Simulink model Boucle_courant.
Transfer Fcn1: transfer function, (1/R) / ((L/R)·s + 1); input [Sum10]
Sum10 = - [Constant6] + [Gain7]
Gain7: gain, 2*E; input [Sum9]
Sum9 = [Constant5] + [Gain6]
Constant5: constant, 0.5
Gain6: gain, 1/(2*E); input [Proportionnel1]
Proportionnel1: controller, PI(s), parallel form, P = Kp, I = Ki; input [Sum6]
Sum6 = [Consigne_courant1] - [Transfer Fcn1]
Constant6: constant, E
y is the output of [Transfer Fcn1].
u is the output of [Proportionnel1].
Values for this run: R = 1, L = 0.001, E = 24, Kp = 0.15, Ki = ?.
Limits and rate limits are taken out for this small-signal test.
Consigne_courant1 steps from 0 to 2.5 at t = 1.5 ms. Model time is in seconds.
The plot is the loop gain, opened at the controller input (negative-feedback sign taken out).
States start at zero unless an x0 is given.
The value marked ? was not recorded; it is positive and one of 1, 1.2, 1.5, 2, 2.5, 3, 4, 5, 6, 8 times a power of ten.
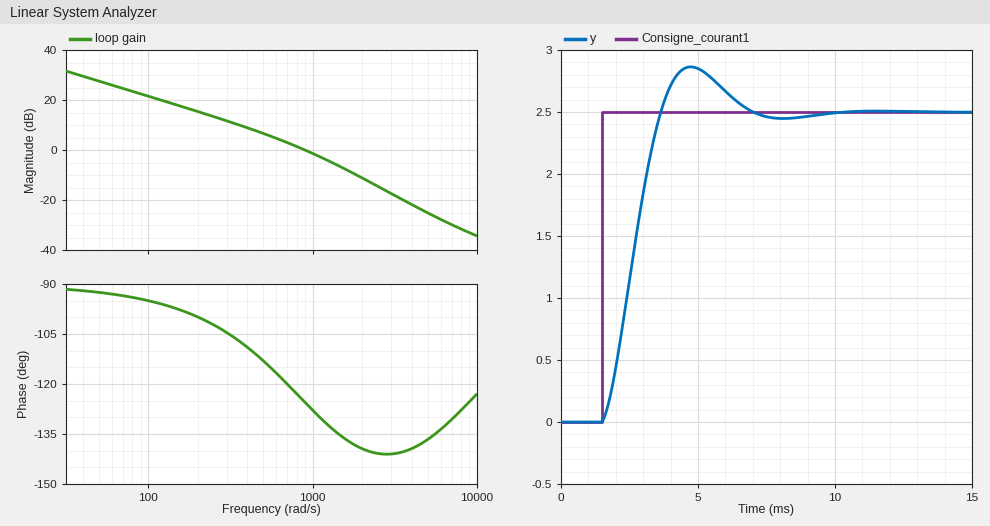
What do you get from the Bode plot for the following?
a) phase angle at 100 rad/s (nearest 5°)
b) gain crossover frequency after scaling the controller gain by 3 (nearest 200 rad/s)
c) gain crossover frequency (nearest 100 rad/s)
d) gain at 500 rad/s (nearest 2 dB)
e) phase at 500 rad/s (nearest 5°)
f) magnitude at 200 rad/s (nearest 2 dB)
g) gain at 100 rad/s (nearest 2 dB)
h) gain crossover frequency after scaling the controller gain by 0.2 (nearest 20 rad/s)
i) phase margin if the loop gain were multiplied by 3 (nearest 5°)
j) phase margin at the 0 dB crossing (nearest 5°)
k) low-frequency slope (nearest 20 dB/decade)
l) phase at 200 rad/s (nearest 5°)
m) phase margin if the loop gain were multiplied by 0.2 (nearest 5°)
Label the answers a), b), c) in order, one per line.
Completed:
a) -95°
b) 1800 rad/s
c) 900 rad/s
d) 6 dB
e) -115°
f) 16 dB
g) 22 dB
h) 240 rad/s
i) 40°
j) 55°
k) -20 dB/decade
l) -100°
m) 80°
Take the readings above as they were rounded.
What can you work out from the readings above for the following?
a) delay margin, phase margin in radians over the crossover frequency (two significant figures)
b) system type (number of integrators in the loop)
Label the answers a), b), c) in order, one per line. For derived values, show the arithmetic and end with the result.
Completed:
a) 55 × π / 180 / 900 = 0.0011 s
b) 1
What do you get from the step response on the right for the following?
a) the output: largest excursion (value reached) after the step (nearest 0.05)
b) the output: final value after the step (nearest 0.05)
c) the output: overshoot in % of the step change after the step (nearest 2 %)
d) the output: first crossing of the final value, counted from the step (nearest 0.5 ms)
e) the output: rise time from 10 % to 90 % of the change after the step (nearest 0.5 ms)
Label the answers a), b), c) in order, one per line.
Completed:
a) 2.85
b) 2.50
c) 14 %
d) 2.0 ms
e) 1.5 ms
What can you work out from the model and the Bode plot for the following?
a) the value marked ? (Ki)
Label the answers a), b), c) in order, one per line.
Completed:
a) 1200
